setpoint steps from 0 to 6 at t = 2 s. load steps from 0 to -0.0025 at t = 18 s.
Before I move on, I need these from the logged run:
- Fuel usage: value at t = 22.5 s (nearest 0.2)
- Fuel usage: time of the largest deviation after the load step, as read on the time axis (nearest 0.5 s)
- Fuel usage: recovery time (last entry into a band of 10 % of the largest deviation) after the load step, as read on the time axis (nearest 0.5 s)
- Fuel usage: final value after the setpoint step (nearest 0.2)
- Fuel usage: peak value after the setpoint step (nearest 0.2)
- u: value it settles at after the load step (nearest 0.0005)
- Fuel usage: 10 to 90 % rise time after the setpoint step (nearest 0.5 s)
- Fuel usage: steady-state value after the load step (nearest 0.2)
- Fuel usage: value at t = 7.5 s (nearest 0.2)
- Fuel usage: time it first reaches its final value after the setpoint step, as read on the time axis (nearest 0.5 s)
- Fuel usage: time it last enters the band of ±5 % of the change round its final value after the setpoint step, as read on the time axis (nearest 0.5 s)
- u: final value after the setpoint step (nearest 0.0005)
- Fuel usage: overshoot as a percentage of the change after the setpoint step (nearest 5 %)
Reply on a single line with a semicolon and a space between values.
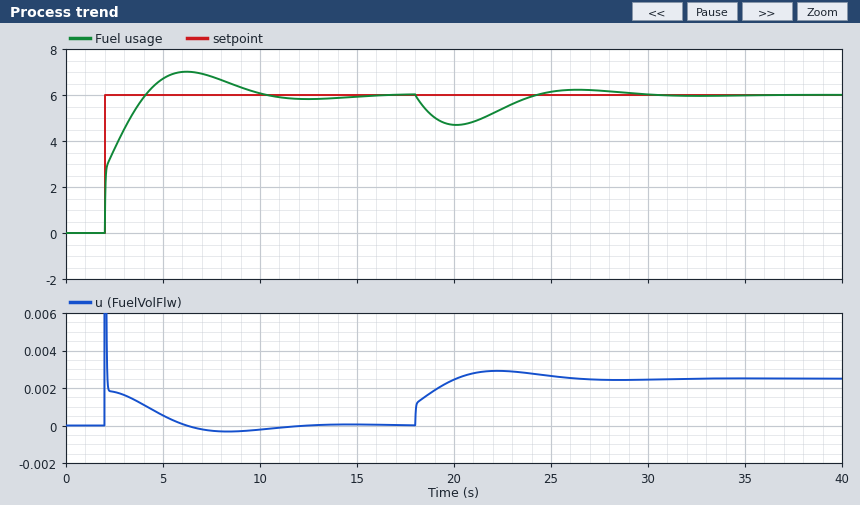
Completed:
5.4; 20.0 s; 28.5 s; 6.0; 7.0; 0.0025; 1.5 s; 6.0; 6.8; 4.0 s; 9.0 s; 0.0000; 15 %
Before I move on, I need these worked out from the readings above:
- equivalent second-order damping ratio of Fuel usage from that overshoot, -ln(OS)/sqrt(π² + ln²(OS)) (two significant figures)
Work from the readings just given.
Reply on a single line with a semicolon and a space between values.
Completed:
0.52
